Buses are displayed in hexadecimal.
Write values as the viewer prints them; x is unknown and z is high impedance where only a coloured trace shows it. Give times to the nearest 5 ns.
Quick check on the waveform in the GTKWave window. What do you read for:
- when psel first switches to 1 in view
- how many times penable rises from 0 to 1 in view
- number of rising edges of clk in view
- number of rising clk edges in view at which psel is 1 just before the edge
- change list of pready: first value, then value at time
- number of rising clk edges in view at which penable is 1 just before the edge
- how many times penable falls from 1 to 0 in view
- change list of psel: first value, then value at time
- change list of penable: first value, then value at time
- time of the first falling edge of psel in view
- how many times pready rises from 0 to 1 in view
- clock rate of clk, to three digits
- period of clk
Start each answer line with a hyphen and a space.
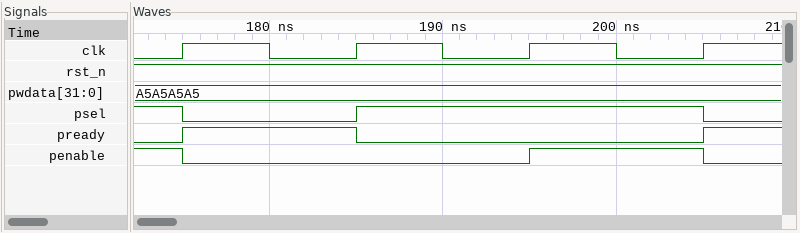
- 185 ns
- 1
- 4
- 3
- 0, 1 at 175 ns, 0 at 185 ns, 1 at 205 ns
- 2
- 2
- 1, 0 at 175 ns, 1 at 185 ns, 0 at 205 ns
- 1, 0 at 175 ns, 1 at 195 ns, 0 at 205 ns
- 175 ns
- 2
- 100 MHz
- 10 ns
